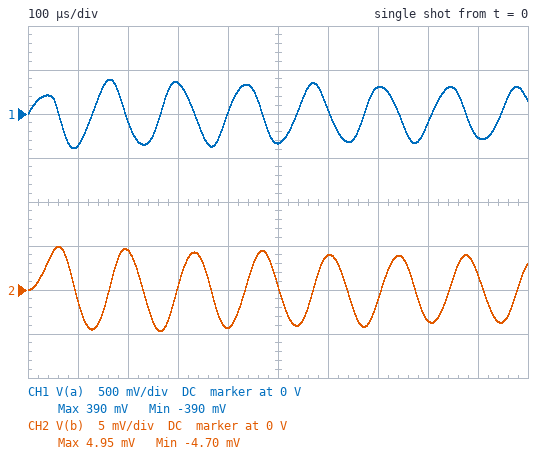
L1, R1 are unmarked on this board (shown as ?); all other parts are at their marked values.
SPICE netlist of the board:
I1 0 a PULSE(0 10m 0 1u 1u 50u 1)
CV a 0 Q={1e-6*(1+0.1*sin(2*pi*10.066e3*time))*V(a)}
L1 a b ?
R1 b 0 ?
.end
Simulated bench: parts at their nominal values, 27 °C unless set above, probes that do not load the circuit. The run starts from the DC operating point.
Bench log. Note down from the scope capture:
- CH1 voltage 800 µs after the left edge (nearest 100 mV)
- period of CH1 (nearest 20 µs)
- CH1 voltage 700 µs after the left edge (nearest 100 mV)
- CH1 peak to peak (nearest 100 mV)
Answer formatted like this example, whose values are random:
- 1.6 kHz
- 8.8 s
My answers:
- -100 mV
- 140 µs
- 300 mV
- 800 mV
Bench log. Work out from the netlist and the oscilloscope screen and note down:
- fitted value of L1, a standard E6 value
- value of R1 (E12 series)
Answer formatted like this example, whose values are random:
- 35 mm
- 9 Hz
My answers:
- 470 µH
- 0.27 Ω
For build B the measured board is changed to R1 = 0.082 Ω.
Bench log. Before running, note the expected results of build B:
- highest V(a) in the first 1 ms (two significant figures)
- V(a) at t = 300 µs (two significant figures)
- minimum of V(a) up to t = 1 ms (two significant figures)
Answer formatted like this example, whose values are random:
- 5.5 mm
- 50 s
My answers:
- 400 mV
- 370 mV
- -400 mV
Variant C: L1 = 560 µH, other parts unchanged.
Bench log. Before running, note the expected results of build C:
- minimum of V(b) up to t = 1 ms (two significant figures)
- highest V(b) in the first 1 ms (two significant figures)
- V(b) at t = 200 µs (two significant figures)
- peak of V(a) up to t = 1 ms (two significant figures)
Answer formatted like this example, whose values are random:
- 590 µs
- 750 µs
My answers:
- -4.5 mV
- 4.7 mV
- 3.8 mV
- 400 mV
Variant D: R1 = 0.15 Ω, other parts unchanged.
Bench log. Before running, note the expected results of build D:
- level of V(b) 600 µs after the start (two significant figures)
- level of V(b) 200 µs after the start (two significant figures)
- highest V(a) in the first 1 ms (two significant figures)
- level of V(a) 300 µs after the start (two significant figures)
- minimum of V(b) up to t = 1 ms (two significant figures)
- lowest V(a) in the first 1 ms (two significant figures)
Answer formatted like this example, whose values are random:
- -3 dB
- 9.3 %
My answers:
- 2.4 mV
- 2.6 mV
- 400 mV
- 370 mV
- -2.7 mV
- -390 mV
